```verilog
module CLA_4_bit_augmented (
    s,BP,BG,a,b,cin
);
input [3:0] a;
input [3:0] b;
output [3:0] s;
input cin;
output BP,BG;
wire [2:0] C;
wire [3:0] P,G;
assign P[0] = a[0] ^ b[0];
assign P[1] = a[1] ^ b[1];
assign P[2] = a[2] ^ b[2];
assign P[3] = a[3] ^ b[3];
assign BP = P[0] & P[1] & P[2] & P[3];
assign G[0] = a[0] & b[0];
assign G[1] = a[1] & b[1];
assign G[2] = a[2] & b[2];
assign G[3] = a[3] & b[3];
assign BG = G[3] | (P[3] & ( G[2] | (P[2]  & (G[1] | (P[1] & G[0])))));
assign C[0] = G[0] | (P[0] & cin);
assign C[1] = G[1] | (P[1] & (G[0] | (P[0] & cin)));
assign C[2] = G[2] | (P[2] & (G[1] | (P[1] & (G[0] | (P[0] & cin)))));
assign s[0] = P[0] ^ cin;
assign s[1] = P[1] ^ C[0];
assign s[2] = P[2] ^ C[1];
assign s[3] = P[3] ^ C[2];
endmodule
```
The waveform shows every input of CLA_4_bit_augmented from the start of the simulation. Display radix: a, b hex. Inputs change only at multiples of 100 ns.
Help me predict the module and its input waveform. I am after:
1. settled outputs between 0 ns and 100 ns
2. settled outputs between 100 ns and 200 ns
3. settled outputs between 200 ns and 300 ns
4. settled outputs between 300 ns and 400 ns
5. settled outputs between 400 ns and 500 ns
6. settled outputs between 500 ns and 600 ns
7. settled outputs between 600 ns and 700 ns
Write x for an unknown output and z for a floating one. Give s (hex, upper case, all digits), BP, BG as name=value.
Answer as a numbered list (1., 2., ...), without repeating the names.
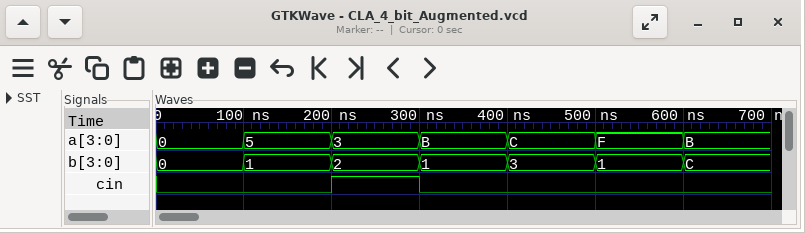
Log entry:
1. s=0, BP=0, BG=0
2. s=6, BP=0, BG=0
3. s=6, BP=0, BG=0
4. s=C, BP=0, BG=0
5. s=F, BP=1, BG=0
6. s=0, BP=0, BG=1
7. s=7, BP=0, BG=1
